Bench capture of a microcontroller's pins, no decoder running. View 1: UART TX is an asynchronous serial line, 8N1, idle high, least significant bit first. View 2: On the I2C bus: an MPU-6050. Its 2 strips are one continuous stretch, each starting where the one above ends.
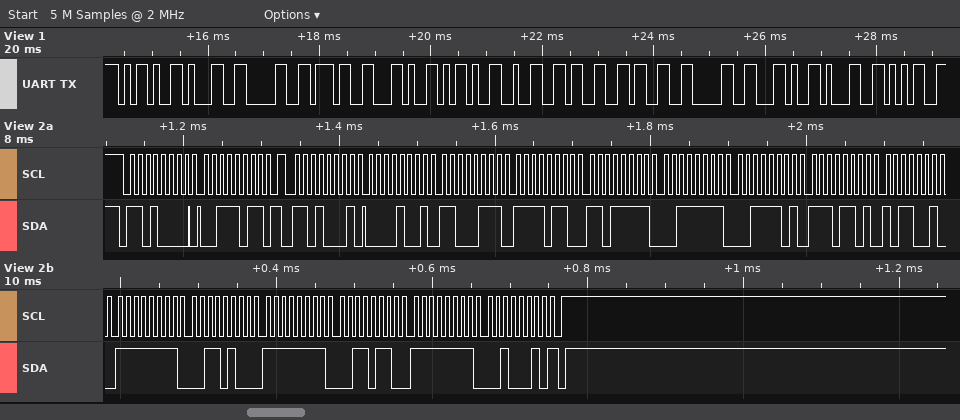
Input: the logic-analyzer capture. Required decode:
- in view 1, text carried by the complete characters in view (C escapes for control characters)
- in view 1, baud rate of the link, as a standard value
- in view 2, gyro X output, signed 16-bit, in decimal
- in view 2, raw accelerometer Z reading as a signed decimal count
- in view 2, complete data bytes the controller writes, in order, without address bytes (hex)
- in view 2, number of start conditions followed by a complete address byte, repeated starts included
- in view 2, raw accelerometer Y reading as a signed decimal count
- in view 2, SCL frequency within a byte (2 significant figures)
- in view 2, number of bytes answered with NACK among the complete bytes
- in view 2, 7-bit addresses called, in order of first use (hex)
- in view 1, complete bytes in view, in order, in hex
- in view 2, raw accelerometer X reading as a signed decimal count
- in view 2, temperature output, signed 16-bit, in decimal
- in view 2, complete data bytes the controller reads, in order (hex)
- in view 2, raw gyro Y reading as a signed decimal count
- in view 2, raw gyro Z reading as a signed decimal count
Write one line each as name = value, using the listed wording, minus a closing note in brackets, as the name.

in view 1, text carried by the complete characters in view = "-107,-2330,15"
in view 1, baud rate of the link, as a standard value = 9600 baud
in view 2, gyro X output, signed 16-bit, in decimal = -204
in view 2, raw accelerometer Z reading as a signed decimal count = 16189
in view 2, complete data bytes the controller writes, in order, without address bytes = 3B
in view 2, number of start conditions followed by a complete address byte, repeated starts included = 2
in view 2, raw accelerometer Y reading as a signed decimal count = -2337
in view 2, SCL frequency within a byte = 100 kHz
in view 2, number of bytes answered with NACK among the complete bytes = 1
in view 2, 7-bit addresses called, in order of first use = 0x68
in view 1, complete bytes in view, in order, in hex = 2D 31 30 37 2C 2D 32 33 33 30 2C 31 35
in view 2, raw accelerometer X reading as a signed decimal count = 2503
in view 2, temperature output, signed 16-bit, in decimal = -4686
in view 2, complete data bytes the controller reads, in order = 09 C7 F6 DF 3F 3D ED B2 FF 34 FF 36 FF 22
in view 2, raw gyro Y reading as a signed decimal count = -202
in view 2, raw gyro Z reading as a signed decimal count = -222
